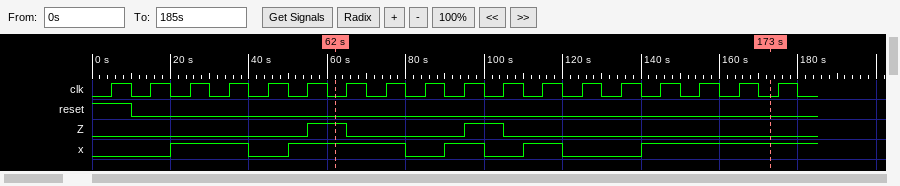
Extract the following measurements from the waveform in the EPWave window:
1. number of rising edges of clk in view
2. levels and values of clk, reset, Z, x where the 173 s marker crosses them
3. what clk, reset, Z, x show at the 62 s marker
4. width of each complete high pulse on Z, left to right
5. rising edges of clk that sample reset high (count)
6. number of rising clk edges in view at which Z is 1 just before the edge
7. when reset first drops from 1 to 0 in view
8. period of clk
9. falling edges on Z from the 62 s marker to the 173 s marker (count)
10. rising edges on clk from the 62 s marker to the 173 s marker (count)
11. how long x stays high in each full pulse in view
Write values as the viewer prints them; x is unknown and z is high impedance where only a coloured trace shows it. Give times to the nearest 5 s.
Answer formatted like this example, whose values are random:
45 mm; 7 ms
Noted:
18; clk=0, reset=0, Z=0, x=1; clk=0, reset=0, Z=1, x=1; 10 s, 10 s; 1; 2; 10 s; 10 s; 2; 11; 20 s, 30 s, 10 s, 10 s
